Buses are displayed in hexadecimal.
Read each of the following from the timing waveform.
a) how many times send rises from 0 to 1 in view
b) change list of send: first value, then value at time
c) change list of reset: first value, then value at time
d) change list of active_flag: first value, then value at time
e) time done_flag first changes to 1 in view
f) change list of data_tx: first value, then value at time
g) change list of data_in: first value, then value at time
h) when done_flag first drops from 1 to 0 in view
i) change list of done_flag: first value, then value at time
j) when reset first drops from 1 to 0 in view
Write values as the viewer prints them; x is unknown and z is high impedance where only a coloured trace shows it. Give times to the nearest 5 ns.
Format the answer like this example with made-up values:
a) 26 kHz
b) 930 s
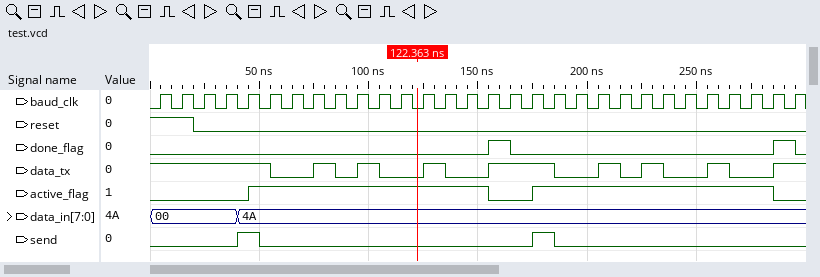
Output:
a) 2
b) 0, 1 at 40 ns, 0 at 50 ns, 1 at 175 ns, 0 at 185 ns
c) 1, 0 at 20 ns
d) 0, 1 at 45 ns, 0 at 155 ns, 1 at 175 ns, 0 at 285 ns
e) 155 ns
f) 1, 0 at 55 ns, 1 at 75 ns, 0 at 85 ns, 1 at 95 ns, 0 at 105 ns, 1 at 125 ns, 0 at 135 ns, 1 at 155 ns, 0 at 185 ns, 1 at 205 ns, 0 at 215 ns, 1 at 225 ns, 0 at 235 ns, 1 at 255 ns, 0 at 265 ns, 1 at 285 ns
g) 00, 4A at 40 ns
h) 165 ns
i) 0, 1 at 155 ns, 0 at 165 ns, 1 at 285 ns, 0 at 295 ns
j) 20 ns
